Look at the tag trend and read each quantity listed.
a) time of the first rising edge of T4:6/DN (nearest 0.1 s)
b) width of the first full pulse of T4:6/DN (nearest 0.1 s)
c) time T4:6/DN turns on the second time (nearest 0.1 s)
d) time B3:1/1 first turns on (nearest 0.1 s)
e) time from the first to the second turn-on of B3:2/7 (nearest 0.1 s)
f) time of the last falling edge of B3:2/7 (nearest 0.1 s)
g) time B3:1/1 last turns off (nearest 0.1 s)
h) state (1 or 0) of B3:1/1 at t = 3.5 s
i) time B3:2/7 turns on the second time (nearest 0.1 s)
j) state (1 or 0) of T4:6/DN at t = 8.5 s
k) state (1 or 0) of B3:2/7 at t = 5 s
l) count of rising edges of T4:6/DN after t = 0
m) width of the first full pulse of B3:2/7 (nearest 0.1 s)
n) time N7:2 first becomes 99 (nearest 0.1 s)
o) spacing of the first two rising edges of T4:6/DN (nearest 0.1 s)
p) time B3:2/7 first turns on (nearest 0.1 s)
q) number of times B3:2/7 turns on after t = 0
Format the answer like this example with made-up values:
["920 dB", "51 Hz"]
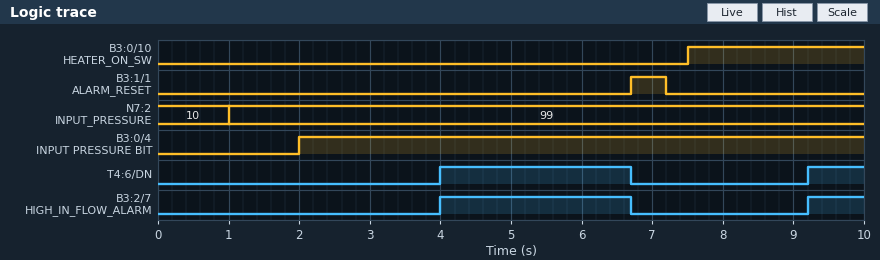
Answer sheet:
["4.0 s", "2.7 s", "9.2 s", "6.7 s", "5.2 s", "6.7 s", "7.2 s", "0", "9.2 s", "0", "1", "2", "2.7 s", "1.0 s", "5.2 s", "4.0 s", "2"]
